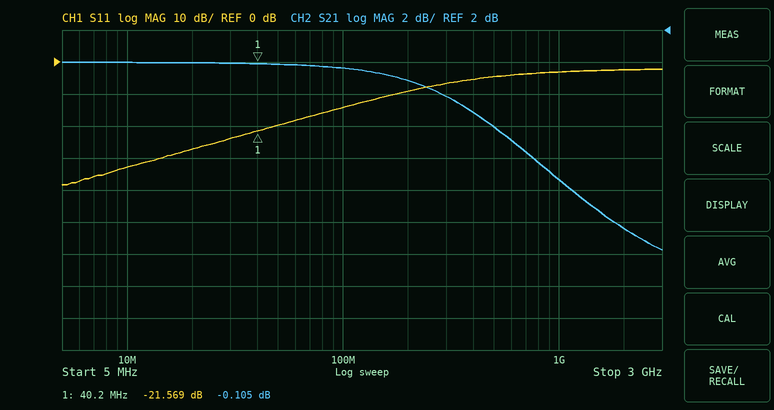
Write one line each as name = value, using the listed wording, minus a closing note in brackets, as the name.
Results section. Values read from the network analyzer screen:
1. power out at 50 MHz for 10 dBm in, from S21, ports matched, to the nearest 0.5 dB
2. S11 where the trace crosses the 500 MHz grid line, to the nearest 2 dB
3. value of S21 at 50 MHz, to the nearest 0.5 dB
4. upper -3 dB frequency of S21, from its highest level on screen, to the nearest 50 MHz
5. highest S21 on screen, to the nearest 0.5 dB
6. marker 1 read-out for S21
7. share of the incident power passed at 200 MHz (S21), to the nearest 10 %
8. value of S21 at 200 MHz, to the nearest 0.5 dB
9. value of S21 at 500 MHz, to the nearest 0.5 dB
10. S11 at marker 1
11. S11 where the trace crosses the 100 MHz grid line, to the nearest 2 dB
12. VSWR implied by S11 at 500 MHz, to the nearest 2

power out at 50 MHz for 10 dBm in, from S21, ports matched, to the nearest 0.5 dB = 10.0 dBm
S11 where the trace crosses the 500 MHz grid line, to the nearest 2 dB = -4 dB
value of S21 at 50 MHz, to the nearest 0.5 dB = 0.0 dB
upper -3 dB frequency of S21, from its highest level on screen, to the nearest 50 MHz = 400 MHz
highest S21 on screen, to the nearest 0.5 dB = 0.0 dB
marker 1 read-out for S21 = -0.105 dB
share of the incident power passed at 200 MHz (S21), to the nearest 10 % = 80 %
value of S21 at 200 MHz, to the nearest 0.5 dB = -1.0 dB
value of S21 at 500 MHz, to the nearest 0.5 dB = -4.0 dB
S11 at marker 1 = -21.569 dB
S11 where the trace crosses the 100 MHz grid line, to the nearest 2 dB = -14 dB
VSWR implied by S11 at 500 MHz, to the nearest 2 = 4
